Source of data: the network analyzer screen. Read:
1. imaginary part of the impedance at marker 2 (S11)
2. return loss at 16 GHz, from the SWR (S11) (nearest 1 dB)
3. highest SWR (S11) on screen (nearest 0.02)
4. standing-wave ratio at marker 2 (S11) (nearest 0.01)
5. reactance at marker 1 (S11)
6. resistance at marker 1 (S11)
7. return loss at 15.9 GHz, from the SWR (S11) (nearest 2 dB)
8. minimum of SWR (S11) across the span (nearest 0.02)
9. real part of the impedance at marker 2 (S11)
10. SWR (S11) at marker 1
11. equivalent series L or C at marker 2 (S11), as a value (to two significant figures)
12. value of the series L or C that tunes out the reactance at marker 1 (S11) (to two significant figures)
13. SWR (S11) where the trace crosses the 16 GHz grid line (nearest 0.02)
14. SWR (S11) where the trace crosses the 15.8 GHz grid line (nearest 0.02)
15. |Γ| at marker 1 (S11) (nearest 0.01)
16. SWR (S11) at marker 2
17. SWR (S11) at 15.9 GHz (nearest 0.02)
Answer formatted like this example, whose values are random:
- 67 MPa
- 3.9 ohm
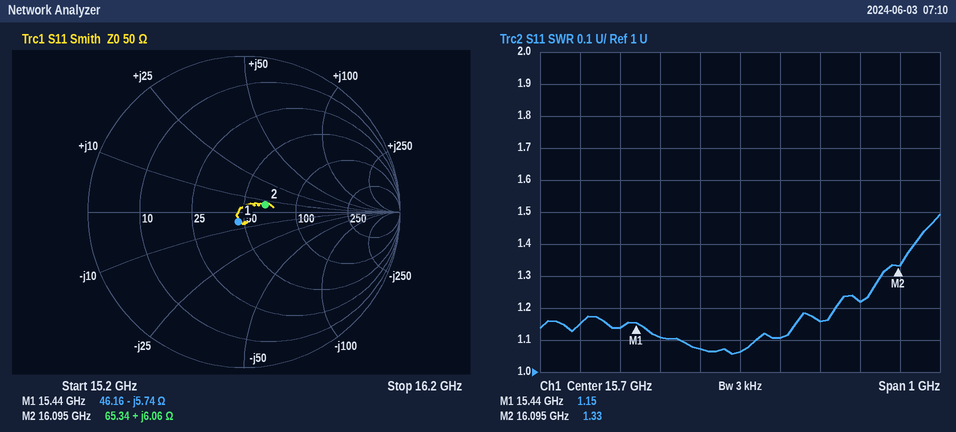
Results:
- +6.06 Ω
- 20 dB
- 1.50
- 1.33
- -5.74 Ω
- 46.16 Ω
- 22 dB
- 1.06
- 65.34 Ω
- 1.15
- 60 pH
- 59 pH
- 1.22
- 1.10
- 0.07
- 1.33
- 1.16
